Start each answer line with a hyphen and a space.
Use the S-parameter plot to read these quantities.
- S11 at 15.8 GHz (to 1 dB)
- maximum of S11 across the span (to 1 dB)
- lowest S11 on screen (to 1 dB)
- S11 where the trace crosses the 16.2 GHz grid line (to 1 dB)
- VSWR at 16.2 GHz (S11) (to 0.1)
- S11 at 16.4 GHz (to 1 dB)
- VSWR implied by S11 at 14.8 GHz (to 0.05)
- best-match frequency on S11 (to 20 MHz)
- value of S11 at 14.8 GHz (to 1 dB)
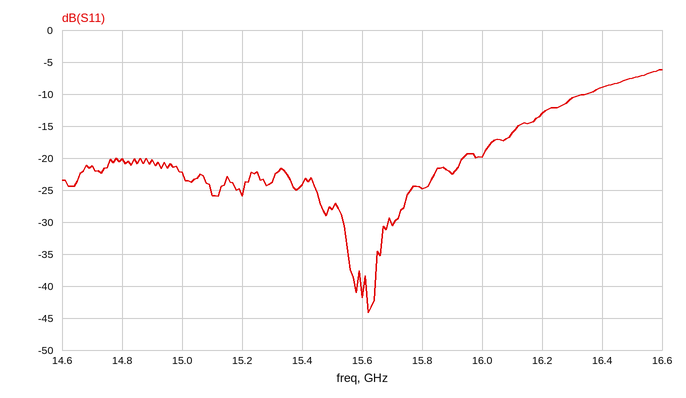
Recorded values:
- -25 dB
- -6 dB
- -44 dB
- -13 dB
- 1.6
- -9 dB
- 1.20
- 15.62 GHz
- -20 dB
